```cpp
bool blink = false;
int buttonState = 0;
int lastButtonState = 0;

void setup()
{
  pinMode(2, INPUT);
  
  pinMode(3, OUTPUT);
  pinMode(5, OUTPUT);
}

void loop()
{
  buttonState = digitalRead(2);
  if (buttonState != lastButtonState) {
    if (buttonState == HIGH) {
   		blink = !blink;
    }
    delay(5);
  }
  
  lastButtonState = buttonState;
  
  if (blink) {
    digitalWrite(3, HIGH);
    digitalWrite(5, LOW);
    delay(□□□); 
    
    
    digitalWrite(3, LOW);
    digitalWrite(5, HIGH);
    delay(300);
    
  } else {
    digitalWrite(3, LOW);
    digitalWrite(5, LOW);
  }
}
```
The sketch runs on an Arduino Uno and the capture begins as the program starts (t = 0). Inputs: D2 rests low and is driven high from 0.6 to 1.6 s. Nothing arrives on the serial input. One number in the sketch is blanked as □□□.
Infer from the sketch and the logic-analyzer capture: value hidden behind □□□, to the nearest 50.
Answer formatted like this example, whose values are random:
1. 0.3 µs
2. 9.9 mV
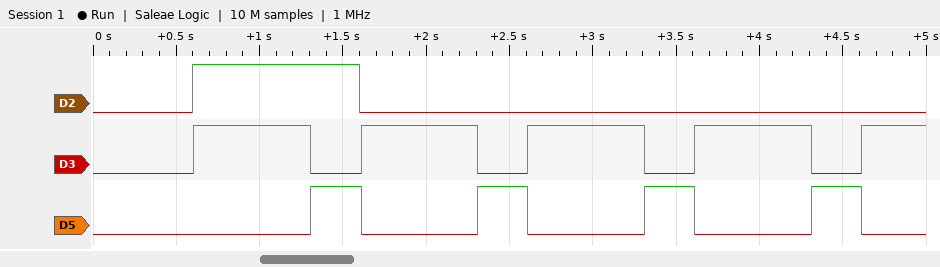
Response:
1. 700
